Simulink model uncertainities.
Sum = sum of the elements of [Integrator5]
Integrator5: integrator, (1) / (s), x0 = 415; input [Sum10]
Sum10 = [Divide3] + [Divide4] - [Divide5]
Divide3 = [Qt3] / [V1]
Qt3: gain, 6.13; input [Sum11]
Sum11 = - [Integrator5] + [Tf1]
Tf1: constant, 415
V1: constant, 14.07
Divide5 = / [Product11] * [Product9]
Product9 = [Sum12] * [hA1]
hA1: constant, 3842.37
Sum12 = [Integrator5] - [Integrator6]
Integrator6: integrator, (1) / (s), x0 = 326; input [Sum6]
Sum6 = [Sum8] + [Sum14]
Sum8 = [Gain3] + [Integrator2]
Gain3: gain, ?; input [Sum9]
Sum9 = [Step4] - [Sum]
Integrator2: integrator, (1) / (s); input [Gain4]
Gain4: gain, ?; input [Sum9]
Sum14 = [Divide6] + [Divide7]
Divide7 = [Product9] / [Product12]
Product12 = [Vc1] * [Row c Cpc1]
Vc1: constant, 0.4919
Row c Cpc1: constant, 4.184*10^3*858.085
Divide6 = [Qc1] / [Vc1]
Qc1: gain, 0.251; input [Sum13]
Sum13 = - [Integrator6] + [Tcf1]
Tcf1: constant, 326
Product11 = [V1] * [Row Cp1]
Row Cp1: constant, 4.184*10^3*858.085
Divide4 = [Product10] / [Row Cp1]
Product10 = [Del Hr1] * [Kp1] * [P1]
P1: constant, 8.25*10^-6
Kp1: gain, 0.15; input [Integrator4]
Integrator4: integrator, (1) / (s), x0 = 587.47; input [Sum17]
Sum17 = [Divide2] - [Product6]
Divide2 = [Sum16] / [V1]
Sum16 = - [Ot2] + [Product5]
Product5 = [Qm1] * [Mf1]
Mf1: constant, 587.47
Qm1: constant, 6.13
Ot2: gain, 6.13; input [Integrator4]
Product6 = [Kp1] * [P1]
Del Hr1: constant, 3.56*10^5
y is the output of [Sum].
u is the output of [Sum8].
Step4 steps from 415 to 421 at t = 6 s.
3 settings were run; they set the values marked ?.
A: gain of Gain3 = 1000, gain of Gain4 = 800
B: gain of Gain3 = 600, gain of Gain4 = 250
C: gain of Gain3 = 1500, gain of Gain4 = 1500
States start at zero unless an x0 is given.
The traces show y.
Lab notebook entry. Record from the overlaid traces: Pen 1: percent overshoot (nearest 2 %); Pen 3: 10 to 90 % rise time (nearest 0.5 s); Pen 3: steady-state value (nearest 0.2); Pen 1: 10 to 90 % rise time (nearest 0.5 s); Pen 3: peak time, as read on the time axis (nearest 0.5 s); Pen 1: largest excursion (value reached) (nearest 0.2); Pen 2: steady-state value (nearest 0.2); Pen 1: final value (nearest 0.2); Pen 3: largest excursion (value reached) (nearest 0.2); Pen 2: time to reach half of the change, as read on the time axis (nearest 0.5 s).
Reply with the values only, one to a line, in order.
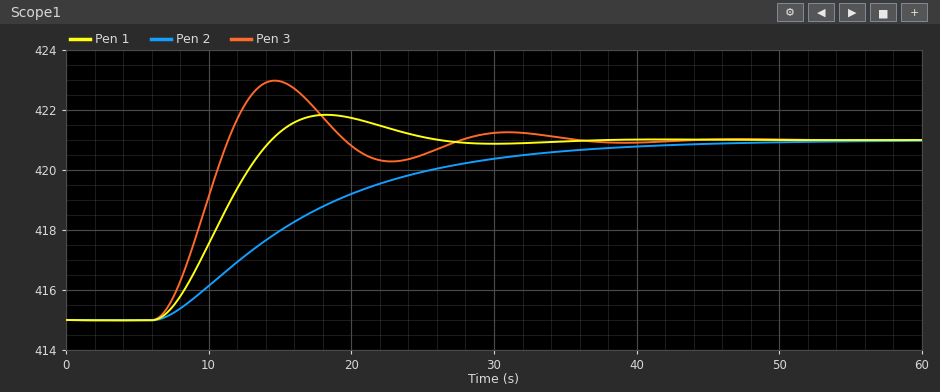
14 %
3.5 s
421.0
5.5 s
14.5 s
421.8
421.0
421.0
423.0
15.0 s
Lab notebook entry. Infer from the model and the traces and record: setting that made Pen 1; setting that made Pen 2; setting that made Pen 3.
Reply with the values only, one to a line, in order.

A
B
C
